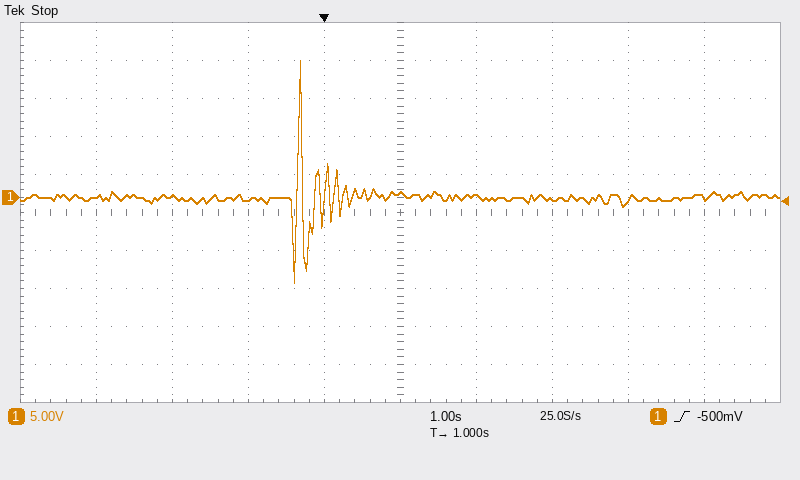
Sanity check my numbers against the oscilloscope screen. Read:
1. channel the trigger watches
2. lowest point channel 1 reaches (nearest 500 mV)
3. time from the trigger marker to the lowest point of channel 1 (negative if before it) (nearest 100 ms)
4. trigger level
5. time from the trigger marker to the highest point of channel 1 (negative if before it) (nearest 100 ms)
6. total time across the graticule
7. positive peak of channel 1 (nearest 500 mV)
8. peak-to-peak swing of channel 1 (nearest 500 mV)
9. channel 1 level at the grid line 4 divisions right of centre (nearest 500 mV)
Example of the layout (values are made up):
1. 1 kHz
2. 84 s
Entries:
1. channel 1
2. -11.0 V
3. -400 ms
4. -500 mV
5. -300 ms
6. 10 s
7. 18.0 V
8. 29.0 V
9. 0.0 V
